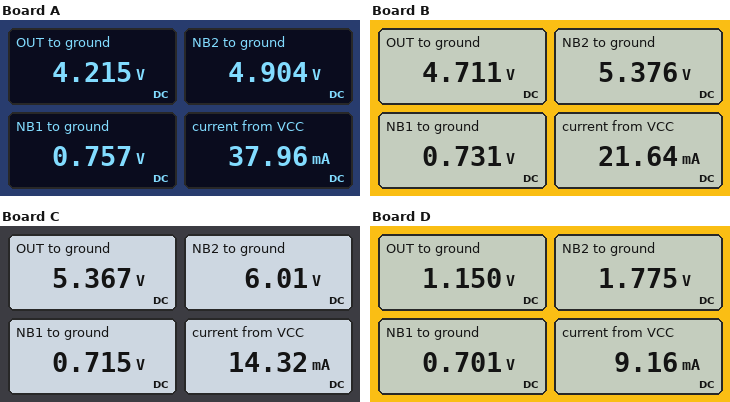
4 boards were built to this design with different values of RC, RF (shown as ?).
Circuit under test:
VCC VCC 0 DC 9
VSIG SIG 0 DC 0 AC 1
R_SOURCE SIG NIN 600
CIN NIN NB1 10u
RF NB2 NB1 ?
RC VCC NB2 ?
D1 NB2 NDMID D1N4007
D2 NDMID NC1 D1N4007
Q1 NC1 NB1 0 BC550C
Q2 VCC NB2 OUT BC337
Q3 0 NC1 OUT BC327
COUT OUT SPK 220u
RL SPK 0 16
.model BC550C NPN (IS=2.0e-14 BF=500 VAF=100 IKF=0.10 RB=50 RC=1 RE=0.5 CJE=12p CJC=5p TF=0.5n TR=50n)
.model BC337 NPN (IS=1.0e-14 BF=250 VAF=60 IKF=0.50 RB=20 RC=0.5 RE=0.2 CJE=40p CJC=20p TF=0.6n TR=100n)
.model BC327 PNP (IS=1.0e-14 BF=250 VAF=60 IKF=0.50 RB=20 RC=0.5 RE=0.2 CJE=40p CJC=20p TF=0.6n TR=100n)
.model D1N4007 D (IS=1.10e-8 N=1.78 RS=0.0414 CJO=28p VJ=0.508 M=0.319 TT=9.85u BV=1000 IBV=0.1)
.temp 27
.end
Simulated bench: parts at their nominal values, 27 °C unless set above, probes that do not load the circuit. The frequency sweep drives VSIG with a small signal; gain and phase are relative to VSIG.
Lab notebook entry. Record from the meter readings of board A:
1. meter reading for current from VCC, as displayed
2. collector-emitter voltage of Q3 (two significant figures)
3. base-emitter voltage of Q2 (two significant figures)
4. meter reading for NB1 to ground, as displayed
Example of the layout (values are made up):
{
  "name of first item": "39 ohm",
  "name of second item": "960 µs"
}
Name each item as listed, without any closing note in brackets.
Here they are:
{
  "meter reading for current from VCC, as displayed": "37.96 mA",
  "collector-emitter voltage of Q3": "-4.2 V",
  "base-emitter voltage of Q2": "690 mV",
  "meter reading for NB1 to ground, as displayed": "0.757 V"
}
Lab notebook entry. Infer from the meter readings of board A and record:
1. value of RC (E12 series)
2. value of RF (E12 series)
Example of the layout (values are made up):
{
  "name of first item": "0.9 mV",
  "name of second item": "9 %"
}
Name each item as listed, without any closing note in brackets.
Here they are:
{
  "value of RC": "120 Ω",
  "value of RF": "47 kΩ"
}
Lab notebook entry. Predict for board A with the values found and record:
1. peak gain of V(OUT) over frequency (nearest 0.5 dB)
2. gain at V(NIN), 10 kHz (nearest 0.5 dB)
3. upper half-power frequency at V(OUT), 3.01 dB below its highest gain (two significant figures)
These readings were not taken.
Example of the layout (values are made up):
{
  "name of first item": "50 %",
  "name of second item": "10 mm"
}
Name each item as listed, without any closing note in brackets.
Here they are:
{
  "peak gain of V(OUT) over frequency": "25.5 dB",
  "gain at V(NIN), 10 kHz": "-10.0 dB",
  "upper half-power frequency at V(OUT), 3.01 dB below its highest gain": "1.3 MHz"
}
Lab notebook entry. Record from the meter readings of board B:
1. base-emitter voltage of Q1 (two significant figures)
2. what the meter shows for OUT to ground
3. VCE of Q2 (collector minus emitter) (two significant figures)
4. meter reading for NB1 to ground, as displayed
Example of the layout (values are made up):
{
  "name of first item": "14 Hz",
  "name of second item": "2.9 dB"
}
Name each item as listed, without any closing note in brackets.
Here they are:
{
  "base-emitter voltage of Q1": "730 mV",
  "what the meter shows for OUT to ground": "4.711 V",
  "VCE of Q2 (collector minus emitter)": "4.3 V",
  "meter reading for NB1 to ground, as displayed": "0.731 V"
}
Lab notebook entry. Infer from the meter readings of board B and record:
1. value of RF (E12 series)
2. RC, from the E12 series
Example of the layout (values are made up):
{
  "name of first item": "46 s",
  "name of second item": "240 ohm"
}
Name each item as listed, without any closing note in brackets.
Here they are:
{
  "value of RF": "100 kΩ",
  "RC, from the E12 series": "180 Ω"
}
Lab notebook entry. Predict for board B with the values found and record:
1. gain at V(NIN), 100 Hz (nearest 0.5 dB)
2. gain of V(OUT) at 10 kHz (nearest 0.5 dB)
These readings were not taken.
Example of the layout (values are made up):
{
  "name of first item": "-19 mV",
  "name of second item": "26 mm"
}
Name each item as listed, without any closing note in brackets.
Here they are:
{
  "gain at V(NIN), 100 Hz": "-6.5 dB",
  "gain of V(OUT) at 10 kHz": "27.5 dB"
}
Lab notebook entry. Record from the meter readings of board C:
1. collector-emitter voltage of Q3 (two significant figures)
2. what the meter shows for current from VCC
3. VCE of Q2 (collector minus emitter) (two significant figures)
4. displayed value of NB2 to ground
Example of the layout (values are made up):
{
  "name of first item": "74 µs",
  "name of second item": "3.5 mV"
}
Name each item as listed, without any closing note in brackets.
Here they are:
{
  "collector-emitter voltage of Q3": "-5.4 V",
  "what the meter shows for current from VCC": "14.32 mA",
  "VCE of Q2 (collector minus emitter)": "3.6 V",
  "displayed value of NB2 to ground": "6.01 V"
}
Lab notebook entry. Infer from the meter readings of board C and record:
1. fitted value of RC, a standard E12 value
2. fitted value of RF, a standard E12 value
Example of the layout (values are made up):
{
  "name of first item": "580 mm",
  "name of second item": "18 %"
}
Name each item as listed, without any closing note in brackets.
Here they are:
{
  "fitted value of RC, a standard E12 value": "220 Ω",
  "fitted value of RF, a standard E12 value": "180 kΩ"
}
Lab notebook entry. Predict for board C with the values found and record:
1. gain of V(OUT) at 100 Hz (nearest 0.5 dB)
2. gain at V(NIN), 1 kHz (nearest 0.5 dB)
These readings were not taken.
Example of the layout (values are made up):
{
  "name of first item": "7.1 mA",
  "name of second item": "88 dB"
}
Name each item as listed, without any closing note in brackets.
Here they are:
{
  "gain of V(OUT) at 100 Hz": "27.0 dB",
  "gain at V(NIN), 1 kHz": "-5.0 dB"
}
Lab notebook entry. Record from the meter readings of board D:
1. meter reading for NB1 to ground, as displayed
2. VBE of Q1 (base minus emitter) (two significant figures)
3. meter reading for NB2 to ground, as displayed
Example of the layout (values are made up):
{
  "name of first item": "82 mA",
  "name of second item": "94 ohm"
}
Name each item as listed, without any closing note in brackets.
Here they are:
{
  "meter reading for NB1 to ground, as displayed": "0.701 V",
  "VBE of Q1 (base minus emitter)": "700 mV",
  "meter reading for NB2 to ground, as displayed": "1.775 V"
}
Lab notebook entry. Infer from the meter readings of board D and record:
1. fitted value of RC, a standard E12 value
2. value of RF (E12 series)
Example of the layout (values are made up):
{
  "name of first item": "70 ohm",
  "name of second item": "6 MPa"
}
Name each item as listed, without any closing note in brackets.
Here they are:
{
  "fitted value of RC, a standard E12 value": "820 Ω",
  "value of RF": "56 kΩ"
}
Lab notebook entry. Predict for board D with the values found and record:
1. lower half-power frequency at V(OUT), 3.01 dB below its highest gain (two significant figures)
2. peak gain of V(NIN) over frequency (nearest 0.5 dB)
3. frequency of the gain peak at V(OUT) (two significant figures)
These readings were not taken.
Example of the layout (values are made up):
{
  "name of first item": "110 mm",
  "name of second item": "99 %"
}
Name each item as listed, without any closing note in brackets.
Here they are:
{
  "lower half-power frequency at V(OUT), 3.01 dB below its highest gain": "7.1 Hz",
  "peak gain of V(NIN) over frequency": "0 dB",
  "frequency of the gain peak at V(OUT)": "18 Hz"
}
